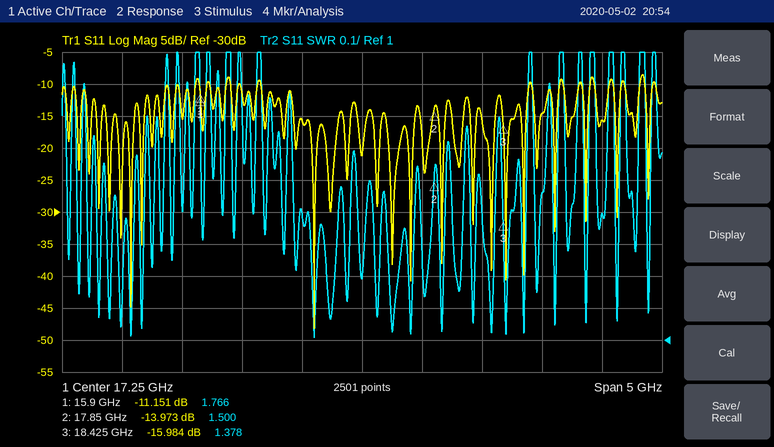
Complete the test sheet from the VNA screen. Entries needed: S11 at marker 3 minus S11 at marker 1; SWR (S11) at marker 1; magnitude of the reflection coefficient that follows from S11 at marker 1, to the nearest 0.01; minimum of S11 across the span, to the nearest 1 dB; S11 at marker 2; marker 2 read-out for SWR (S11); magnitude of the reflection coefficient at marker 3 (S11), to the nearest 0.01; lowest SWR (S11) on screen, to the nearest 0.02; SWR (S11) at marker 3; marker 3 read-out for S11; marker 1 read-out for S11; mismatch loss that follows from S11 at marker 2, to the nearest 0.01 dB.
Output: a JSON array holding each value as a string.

["-4.833 dB", "1.766", "0.28", "-48 dB", "-13.973 dB", "1.500", "0.16", "1.00", "1.378", "-15.984 dB", "-11.151 dB", "0.18 dB"]
